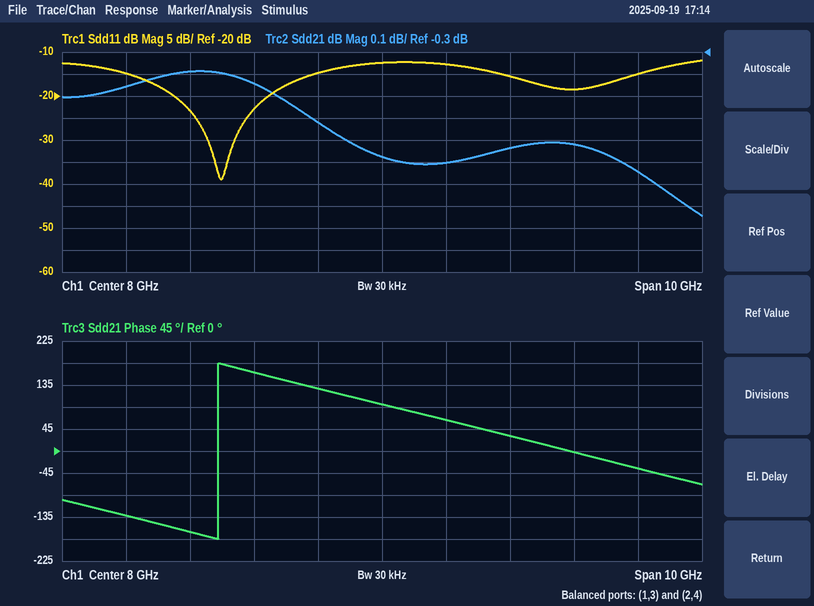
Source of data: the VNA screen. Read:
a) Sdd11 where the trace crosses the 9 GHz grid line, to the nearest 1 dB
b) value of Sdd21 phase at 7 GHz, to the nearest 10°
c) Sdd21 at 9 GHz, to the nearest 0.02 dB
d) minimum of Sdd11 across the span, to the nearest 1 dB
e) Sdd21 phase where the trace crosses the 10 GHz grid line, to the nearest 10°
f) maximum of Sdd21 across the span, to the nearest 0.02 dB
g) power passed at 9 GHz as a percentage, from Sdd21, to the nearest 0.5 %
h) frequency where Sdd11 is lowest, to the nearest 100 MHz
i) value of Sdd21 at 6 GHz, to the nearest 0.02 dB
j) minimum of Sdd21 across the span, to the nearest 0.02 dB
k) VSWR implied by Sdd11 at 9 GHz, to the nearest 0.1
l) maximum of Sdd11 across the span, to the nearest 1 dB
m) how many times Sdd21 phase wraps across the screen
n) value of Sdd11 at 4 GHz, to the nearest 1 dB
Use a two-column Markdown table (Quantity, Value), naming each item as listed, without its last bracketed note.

| Quantity | Value |
|---|---|
| Sdd11 where the trace crosses the 9 GHz grid line, to the nearest 1 dB | -13 dB |
| value of Sdd21 phase at 7 GHz, to the nearest 10° | 130° |
| Sdd21 at 9 GHz, to the nearest 0.02 dB | -0.80 dB |
| minimum of Sdd11 across the span, to the nearest 1 dB | -39 dB |
| Sdd21 phase where the trace crosses the 10 GHz grid line, to the nearest 10° | 30° |
| maximum of Sdd21 across the span, to the nearest 0.02 dB | -0.38 dB |
| power passed at 9 GHz as a percentage, from Sdd21, to the nearest 0.5 % | 83.0 % |
| frequency where Sdd11 is lowest, to the nearest 100 MHz | 5.5 GHz |
| value of Sdd21 at 6 GHz, to the nearest 0.02 dB | -0.44 dB |
| minimum of Sdd21 across the span, to the nearest 0.02 dB | -1.04 dB |
| VSWR implied by Sdd11 at 9 GHz, to the nearest 0.1 | 1.6 |
| maximum of Sdd11 across the span, to the nearest 1 dB | -12 dB |
| how many times Sdd21 phase wraps across the screen | 1 |
| value of Sdd11 at 4 GHz, to the nearest 1 dB | -15 dB |
